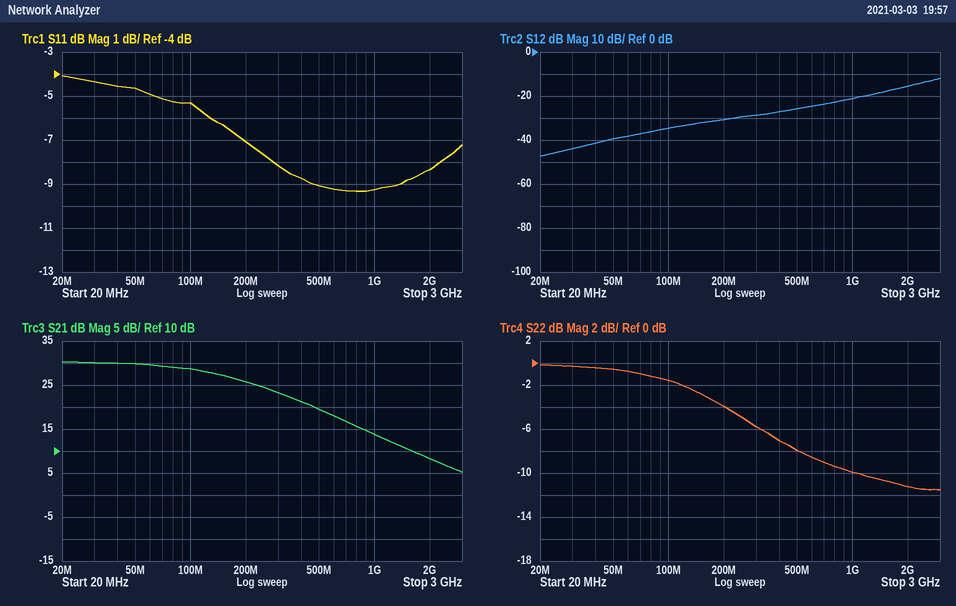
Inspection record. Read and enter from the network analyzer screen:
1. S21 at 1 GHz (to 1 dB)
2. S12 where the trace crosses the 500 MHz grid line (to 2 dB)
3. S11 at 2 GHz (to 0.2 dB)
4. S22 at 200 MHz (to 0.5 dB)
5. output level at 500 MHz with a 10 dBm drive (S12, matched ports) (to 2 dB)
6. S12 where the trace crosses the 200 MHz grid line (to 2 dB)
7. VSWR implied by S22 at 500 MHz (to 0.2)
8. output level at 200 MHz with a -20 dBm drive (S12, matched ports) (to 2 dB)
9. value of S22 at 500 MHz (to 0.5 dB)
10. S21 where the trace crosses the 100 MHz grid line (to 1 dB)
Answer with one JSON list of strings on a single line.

["14 dB", "-26 dB", "-8.4 dB", "-4.0 dB", "-16 dBm", "-30 dB", "2.4", "-50 dBm", "-8.0 dB", "29 dB"]
